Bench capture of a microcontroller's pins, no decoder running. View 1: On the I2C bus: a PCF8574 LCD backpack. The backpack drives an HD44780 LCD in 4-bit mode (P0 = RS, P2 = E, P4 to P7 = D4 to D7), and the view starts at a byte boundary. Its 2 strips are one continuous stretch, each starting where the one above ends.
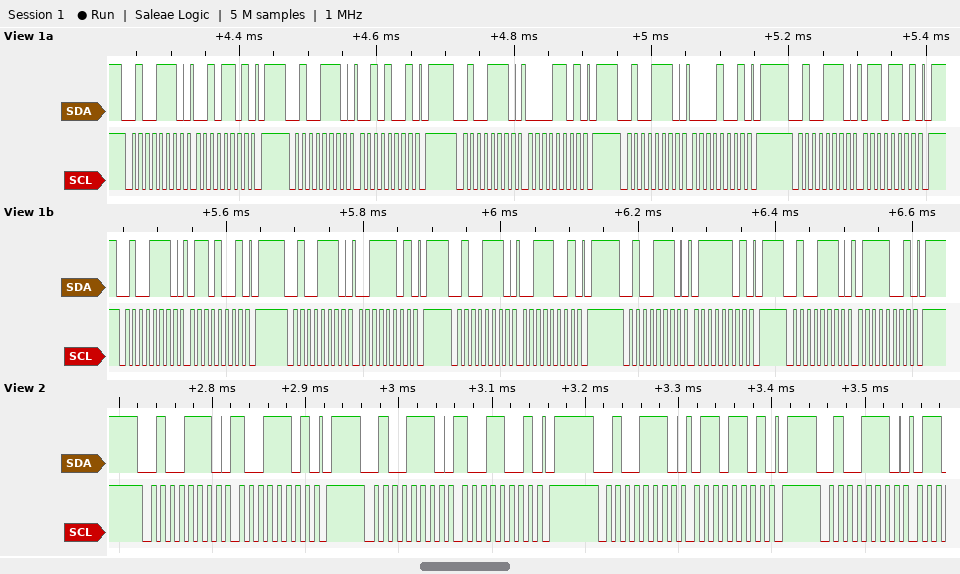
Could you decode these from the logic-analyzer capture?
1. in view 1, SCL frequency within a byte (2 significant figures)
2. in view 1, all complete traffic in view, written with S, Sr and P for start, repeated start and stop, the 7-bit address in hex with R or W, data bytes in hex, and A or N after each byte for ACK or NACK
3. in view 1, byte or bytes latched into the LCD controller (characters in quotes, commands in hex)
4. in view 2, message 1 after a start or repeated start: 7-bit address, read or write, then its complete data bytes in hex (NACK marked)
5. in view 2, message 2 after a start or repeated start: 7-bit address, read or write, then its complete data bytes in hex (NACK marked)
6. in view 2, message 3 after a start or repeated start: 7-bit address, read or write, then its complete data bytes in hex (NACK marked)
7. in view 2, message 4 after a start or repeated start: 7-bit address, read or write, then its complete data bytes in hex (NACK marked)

100 kHz
S 27W A 2D A P S 27W A 29 A P S 27W A 0D A P S 27W A 09 A P S 27W A 6D A P S 27W A 69 A P S 27W A 3D A P S 27W A 39 A P S 27W A 7D A P S 27W A 79 A P
' ' 'c'
0x27 write: 9D
0x27 write: 99
0x27 write: 6D
0x27 write
